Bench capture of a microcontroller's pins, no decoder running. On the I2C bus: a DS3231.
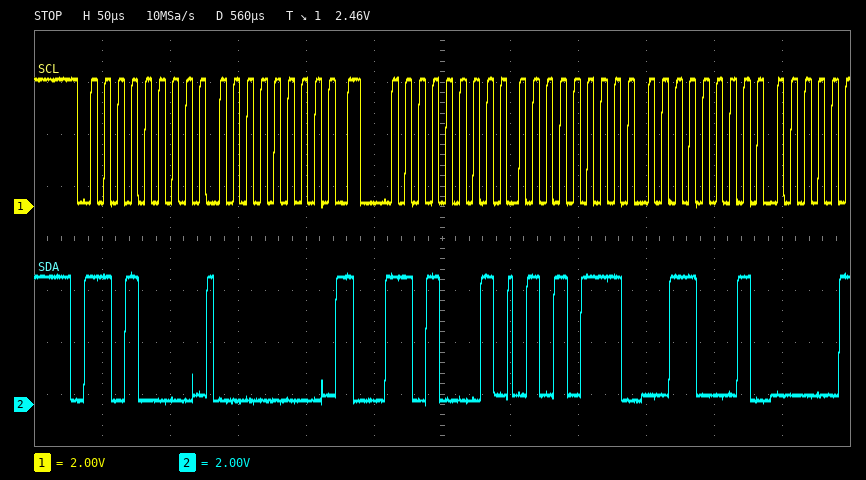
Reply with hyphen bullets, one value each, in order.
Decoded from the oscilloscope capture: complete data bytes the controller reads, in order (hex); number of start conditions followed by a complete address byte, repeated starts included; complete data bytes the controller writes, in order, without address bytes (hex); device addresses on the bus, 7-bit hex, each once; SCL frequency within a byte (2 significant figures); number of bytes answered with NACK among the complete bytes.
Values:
- 57 31
- 2
- 00
- 0x68
- 100 kHz
- 0
